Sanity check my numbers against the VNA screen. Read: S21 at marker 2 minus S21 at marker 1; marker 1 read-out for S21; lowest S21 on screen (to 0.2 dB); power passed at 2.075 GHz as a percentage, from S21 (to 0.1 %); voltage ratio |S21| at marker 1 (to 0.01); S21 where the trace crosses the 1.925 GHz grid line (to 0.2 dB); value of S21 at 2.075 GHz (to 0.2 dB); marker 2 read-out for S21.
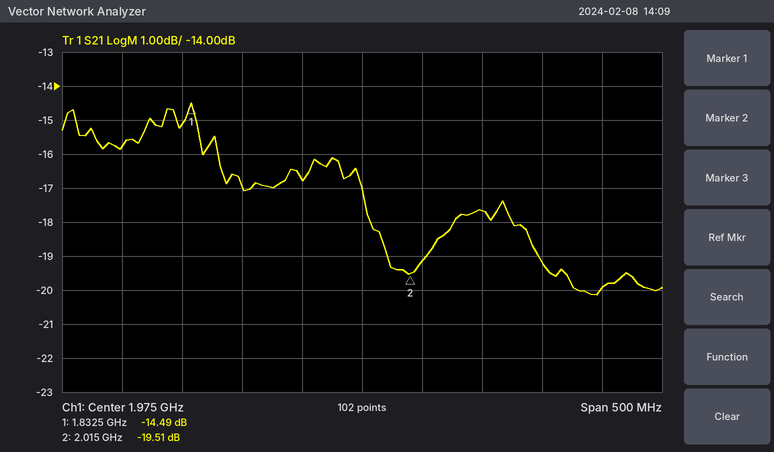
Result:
-5.02 dB
-14.49 dB
-20.2 dB
1.7 %
0.19
-16.8 dB
-17.6 dB
-19.51 dB
